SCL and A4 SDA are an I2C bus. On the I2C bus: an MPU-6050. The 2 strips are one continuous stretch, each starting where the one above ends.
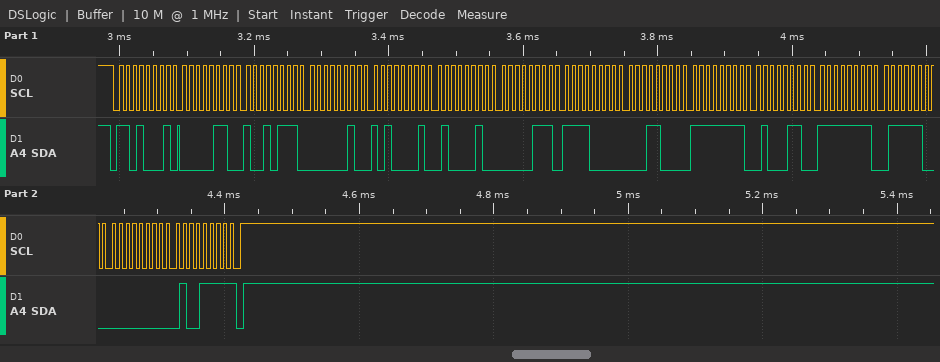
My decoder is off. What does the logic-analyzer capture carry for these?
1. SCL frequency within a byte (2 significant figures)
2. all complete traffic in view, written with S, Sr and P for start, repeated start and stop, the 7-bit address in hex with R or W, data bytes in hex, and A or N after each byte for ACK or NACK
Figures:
100 kHz
S 68R A 06 A 97 A 02 A A1 A 42 A 07 A F0 A 18 A FF A 46 A FF A 7C A 00 A 4F N P
